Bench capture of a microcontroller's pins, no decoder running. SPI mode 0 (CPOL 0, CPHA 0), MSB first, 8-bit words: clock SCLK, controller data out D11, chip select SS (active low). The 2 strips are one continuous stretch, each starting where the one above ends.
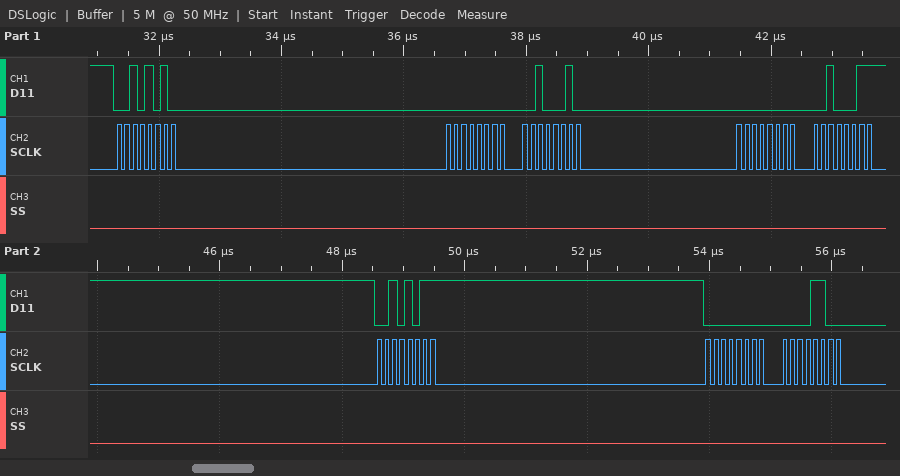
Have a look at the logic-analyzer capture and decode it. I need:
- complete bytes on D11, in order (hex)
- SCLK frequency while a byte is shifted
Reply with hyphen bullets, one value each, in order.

- 2A 00 22 00 23 2B 00 0C
- 8 MHz
